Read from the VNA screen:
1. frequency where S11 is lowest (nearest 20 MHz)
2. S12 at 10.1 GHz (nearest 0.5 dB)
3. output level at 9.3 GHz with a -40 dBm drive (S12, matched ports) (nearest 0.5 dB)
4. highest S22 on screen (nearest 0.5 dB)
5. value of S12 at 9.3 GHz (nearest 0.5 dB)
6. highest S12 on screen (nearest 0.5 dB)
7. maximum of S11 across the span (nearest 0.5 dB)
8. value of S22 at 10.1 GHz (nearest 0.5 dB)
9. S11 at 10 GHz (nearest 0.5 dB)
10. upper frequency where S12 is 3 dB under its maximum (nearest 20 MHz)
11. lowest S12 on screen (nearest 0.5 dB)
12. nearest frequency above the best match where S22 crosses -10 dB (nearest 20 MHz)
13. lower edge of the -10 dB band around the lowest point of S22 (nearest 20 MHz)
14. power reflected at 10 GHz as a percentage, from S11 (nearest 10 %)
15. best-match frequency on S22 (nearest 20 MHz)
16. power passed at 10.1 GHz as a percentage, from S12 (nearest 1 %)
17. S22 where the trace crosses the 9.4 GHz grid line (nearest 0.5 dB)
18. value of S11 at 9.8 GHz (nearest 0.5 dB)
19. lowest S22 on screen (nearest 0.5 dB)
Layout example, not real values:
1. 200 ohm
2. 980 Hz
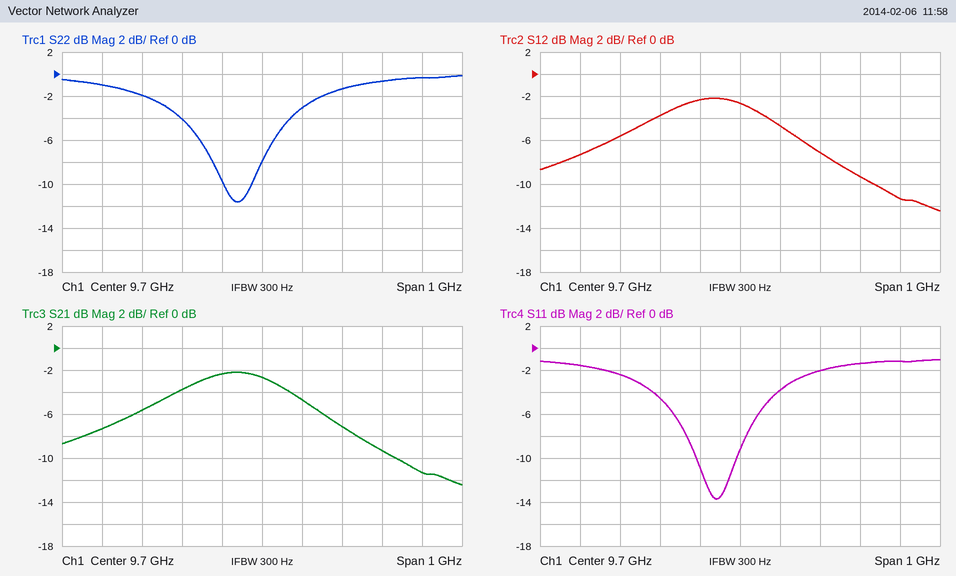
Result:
1. 9.64 GHz
2. -11.5 dB
3. -47.5 dBm
4. 0.0 dB
5. -7.5 dB
6. -2.0 dB
7. -1.0 dB
8. -0.5 dB
9. -1.5 dB
10. 9.82 GHz
11. -12.5 dB
12. 9.68 GHz
13. 9.60 GHz
14. 70 %
15. 9.64 GHz
16. 7 %
17. -2.0 dB
18. -4.0 dB
19. -11.5 dB
